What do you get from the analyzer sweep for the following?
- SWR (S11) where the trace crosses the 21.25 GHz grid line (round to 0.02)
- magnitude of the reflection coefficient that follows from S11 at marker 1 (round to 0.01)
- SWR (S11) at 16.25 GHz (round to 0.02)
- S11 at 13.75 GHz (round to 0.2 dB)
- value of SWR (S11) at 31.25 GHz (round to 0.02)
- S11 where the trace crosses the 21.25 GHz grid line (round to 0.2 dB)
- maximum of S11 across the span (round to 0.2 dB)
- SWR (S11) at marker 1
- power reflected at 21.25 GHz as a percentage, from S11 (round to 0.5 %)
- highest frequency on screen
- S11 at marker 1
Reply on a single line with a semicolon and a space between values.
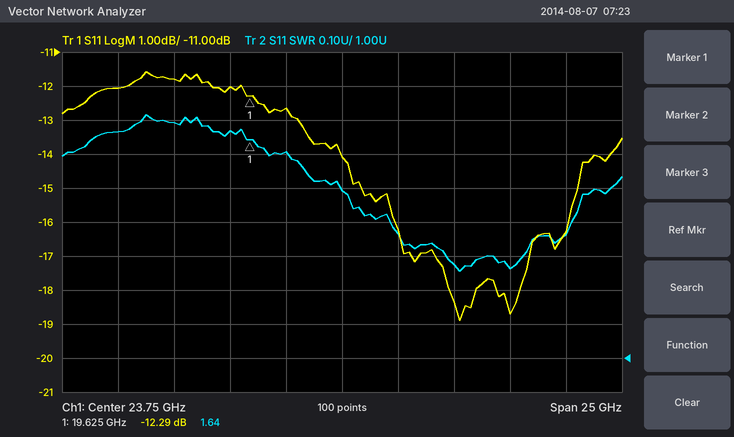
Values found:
1.60; 0.24; 1.70; -12.0 dB; 1.26; -12.6 dB; -11.6 dB; 1.64; 5.5 %; 36.25 GHz; -12.29 dB
